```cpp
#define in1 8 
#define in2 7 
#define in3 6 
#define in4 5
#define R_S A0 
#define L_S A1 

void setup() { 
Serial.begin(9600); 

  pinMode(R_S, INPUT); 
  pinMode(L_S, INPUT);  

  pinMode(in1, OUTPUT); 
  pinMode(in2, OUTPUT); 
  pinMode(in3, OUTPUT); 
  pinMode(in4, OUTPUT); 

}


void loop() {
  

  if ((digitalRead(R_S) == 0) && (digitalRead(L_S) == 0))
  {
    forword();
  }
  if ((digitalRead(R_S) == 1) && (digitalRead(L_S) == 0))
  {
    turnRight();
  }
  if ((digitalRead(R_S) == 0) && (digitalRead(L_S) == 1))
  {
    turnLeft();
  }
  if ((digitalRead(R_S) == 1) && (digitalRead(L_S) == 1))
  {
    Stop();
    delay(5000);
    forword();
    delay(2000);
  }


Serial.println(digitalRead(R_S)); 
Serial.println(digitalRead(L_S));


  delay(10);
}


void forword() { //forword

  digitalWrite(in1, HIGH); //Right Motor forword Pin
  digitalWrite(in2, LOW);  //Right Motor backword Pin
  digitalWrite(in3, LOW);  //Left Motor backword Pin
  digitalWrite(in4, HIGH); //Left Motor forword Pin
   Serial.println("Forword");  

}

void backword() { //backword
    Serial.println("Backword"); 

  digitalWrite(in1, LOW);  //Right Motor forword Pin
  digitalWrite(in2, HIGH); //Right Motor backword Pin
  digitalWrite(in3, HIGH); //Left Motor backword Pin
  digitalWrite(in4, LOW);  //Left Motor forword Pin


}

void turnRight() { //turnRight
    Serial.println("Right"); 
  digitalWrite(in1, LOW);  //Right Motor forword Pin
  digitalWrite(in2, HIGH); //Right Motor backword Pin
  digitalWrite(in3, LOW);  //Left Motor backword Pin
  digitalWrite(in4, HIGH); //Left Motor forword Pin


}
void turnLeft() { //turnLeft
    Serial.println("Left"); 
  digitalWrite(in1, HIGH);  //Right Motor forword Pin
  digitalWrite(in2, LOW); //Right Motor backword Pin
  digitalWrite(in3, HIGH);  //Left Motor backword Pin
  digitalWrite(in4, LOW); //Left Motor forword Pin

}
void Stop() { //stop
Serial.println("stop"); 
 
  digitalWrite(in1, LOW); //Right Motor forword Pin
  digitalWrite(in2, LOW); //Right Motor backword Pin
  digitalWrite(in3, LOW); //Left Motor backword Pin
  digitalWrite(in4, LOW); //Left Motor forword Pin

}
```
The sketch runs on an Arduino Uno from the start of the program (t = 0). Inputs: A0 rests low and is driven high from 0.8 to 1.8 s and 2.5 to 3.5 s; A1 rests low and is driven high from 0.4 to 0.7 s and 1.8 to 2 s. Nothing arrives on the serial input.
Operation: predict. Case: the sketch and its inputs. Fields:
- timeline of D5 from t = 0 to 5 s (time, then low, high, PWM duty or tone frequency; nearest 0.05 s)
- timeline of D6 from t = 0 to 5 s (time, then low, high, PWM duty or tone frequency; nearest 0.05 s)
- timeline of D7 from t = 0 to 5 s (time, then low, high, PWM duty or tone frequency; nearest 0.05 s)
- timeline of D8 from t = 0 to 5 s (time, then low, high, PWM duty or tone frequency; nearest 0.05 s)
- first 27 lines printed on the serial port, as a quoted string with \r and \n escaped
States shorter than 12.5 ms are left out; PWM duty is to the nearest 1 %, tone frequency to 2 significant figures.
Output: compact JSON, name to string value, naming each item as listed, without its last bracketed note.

{"timeline of D5 from t = 0 to 5 s": "0 s high; 0.4 s low; 0.7 s high; 1.8 s low; 2 s high", "timeline of D6 from t = 0 to 5 s": "0 s low; 0.4 s high; 0.7 s low; 1.8 s high; 2 s low", "timeline of D7 from t = 0 to 5 s": "0 s low; 0.8 s high; 1.8 s low; 2.5 s high; 3.5 s low", "timeline of D8 from t = 0 to 5 s": "0 s high; 0.8 s low; 1.8 s high; 2.5 s low; 3.5 s high", "first 27 lines printed on the serial port, as a quoted string with \\r and \\n escaped": "\"Forword\\r\\n0\\r\\n0\\r\\nForword\\r\\n0\\r\\n0\\r\\nForword\\r\\n0\\r\\n0\\r\\nForword\\r\\n0\\r\\n0\\r\\nForword\\r\\n0\\r\\n0\\r\\nForword\\r\\n0\\r\\n0\\r\\nForword\\r\\n0\\r\\n0\\r\\nForword\\r\\n0\\r\\n0\\r\\nForword\\r\\n0\\r\\n0\\r\\n\""}
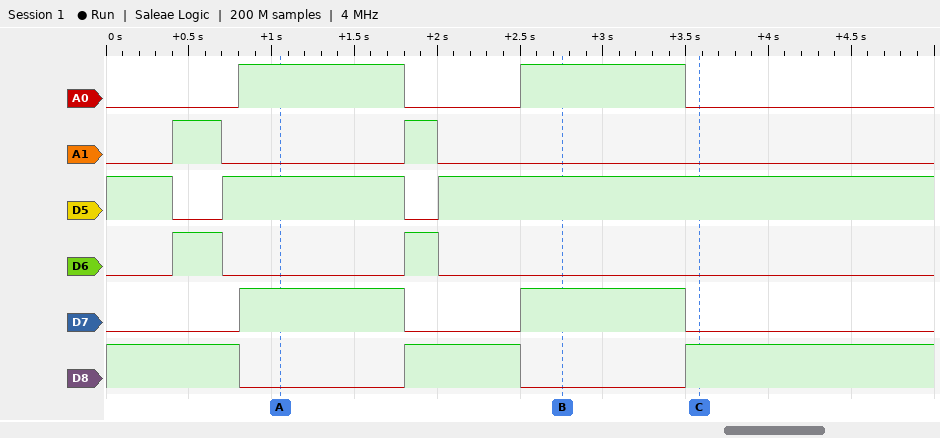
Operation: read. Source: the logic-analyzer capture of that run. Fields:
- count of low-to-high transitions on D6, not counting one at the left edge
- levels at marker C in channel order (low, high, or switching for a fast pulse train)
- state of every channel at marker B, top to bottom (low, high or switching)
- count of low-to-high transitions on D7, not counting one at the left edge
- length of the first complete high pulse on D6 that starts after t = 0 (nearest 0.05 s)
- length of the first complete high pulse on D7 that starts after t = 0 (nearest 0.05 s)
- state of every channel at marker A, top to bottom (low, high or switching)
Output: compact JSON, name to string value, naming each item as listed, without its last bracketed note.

{"count of low-to-high transitions on D6, not counting one at the left edge": "2", "levels at marker C in channel order": "A0 low, A1 low, D5 high, D6 low, D7 low, D8 high", "state of every channel at marker B, top to bottom": "A0 high, A1 low, D5 high, D6 low, D7 high, D8 low", "count of low-to-high transitions on D7, not counting one at the left edge": "2", "length of the first complete high pulse on D6 that starts after t = 0": "0.30 s", "length of the first complete high pulse on D7 that starts after t = 0": "1.00 s", "state of every channel at marker A, top to bottom": "A0 high, A1 low, D5 high, D6 low, D7 high, D8 low"}
